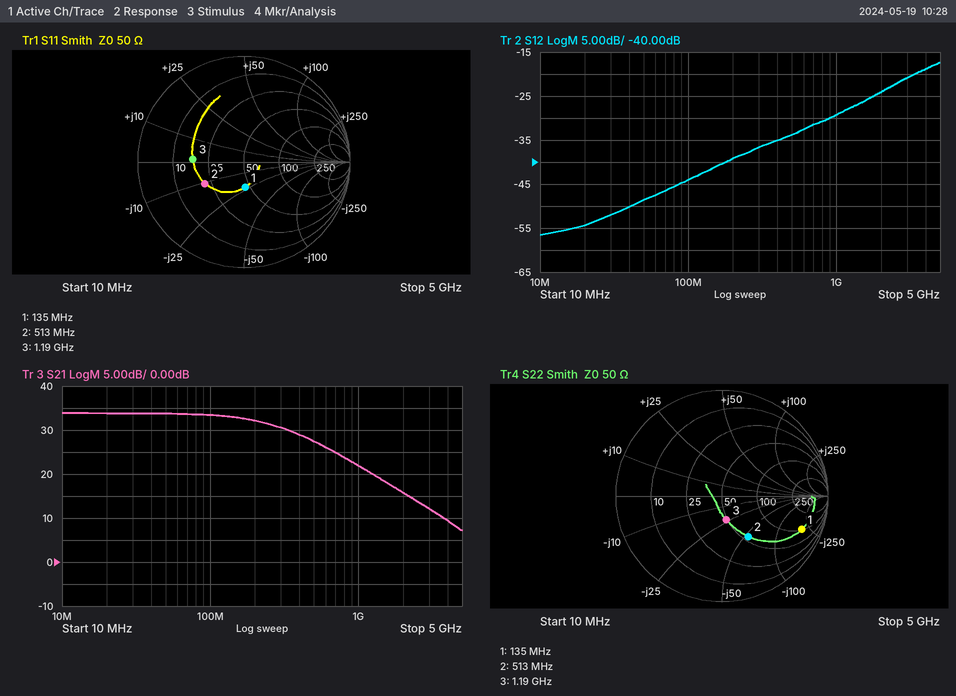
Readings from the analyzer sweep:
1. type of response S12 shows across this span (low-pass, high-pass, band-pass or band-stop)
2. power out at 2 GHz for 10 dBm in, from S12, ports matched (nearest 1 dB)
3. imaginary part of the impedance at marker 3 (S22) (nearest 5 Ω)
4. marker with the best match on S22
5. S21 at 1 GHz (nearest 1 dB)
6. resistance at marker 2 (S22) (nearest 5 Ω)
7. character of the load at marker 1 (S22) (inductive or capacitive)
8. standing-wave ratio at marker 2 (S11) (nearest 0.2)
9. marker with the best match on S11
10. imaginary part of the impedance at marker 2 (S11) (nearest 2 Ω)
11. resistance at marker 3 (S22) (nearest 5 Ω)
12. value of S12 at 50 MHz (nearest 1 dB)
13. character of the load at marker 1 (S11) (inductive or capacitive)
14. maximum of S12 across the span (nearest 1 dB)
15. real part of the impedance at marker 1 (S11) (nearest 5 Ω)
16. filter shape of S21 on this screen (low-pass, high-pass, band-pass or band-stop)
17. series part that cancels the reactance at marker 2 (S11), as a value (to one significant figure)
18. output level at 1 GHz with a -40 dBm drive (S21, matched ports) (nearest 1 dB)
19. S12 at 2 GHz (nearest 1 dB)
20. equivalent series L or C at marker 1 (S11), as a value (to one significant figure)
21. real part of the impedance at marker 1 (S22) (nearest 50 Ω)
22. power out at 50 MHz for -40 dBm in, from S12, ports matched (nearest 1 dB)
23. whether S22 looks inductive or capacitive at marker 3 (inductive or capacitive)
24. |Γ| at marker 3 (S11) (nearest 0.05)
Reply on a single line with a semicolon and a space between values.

high-pass; -14 dBm; -25 Ω; marker 3; 22 dB; 55 Ω; capacitive; 2.4; marker 1; -10 Ω; 50 Ω; -49 dB; capacitive; -17 dB; 45 Ω; low-pass; 3 nH; -18 dBm; -24 dB; 50 pF; 100 Ω; -89 dBm; capacitive; 0.50
